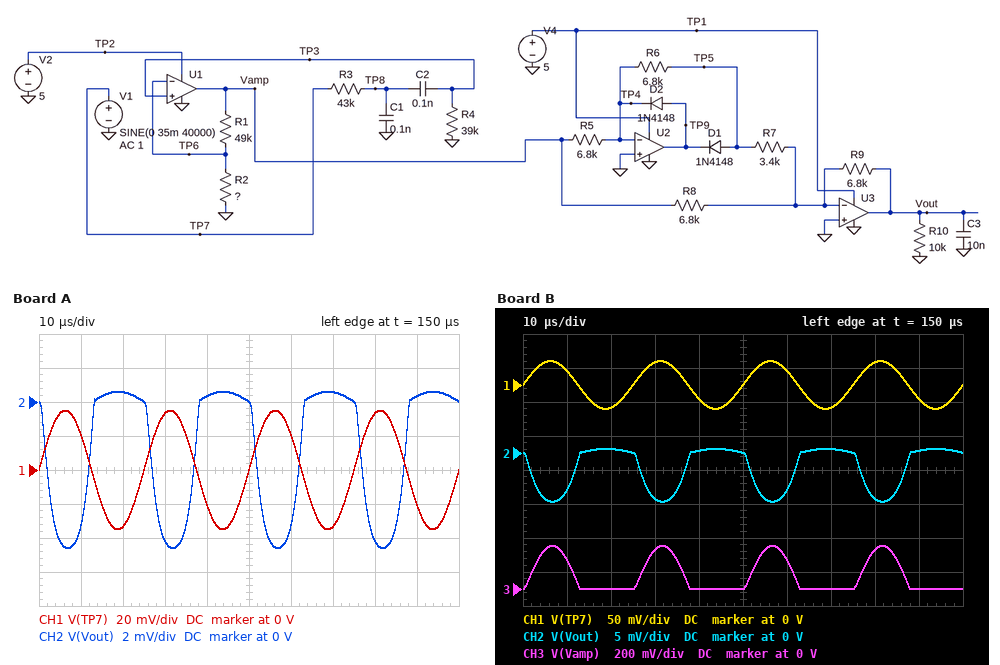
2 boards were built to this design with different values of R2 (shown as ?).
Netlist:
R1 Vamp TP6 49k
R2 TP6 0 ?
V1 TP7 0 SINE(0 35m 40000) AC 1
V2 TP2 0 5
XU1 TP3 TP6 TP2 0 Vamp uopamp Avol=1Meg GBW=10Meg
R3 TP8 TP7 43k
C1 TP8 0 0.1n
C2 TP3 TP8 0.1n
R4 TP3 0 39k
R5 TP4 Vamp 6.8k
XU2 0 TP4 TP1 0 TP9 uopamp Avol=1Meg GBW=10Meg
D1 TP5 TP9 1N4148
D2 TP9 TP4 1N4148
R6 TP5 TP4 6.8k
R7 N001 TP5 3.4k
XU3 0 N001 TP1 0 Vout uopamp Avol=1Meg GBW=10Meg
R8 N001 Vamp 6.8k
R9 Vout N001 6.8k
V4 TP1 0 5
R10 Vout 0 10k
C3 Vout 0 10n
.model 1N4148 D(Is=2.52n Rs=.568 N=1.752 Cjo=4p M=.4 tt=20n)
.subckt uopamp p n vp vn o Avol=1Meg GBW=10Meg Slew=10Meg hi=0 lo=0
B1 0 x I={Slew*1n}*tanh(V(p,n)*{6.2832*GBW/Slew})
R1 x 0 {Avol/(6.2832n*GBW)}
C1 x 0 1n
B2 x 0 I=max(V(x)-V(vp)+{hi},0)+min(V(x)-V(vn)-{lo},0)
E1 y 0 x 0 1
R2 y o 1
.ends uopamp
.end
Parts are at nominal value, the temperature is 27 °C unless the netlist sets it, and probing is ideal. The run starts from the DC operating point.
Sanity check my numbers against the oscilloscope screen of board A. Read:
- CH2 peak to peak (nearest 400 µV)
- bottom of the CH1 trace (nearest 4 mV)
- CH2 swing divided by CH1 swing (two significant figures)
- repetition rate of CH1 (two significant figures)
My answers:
9.2 mV
-36 mV
0.13
40 kHz
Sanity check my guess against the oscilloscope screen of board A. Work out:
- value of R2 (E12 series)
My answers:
1.5 kΩ
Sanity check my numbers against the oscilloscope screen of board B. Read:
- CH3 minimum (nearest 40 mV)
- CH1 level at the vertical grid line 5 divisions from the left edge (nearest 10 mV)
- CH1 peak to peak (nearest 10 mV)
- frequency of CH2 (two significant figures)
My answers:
0 V
0 V
70 mV
40 kHz
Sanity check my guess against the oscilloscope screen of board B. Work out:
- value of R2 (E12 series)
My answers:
2.2 kΩ
